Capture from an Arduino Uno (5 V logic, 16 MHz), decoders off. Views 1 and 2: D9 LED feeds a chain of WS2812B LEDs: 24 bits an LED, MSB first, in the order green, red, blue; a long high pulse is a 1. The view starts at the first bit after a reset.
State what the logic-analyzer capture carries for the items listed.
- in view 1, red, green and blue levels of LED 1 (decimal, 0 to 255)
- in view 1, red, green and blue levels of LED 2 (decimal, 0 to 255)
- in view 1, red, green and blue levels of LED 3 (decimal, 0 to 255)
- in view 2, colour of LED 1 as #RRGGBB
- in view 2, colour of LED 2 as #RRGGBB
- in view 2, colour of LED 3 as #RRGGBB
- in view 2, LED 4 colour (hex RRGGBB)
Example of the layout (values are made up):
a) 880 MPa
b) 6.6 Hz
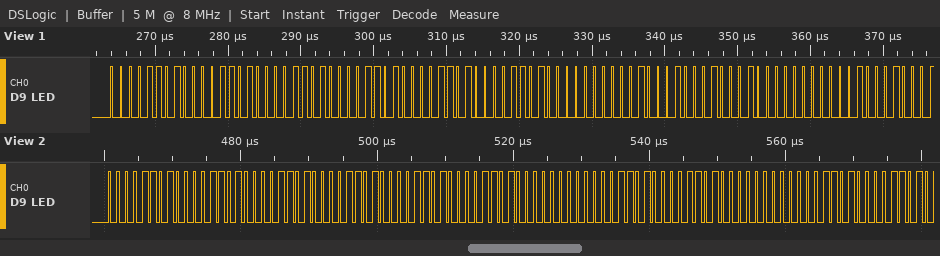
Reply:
a) 13, 13, 13
b) 13, 13, 13
c) 34, 0, 34
d) #0D0D0D
e) #0D0D0D
f) #0D000D
g) #0D000D
